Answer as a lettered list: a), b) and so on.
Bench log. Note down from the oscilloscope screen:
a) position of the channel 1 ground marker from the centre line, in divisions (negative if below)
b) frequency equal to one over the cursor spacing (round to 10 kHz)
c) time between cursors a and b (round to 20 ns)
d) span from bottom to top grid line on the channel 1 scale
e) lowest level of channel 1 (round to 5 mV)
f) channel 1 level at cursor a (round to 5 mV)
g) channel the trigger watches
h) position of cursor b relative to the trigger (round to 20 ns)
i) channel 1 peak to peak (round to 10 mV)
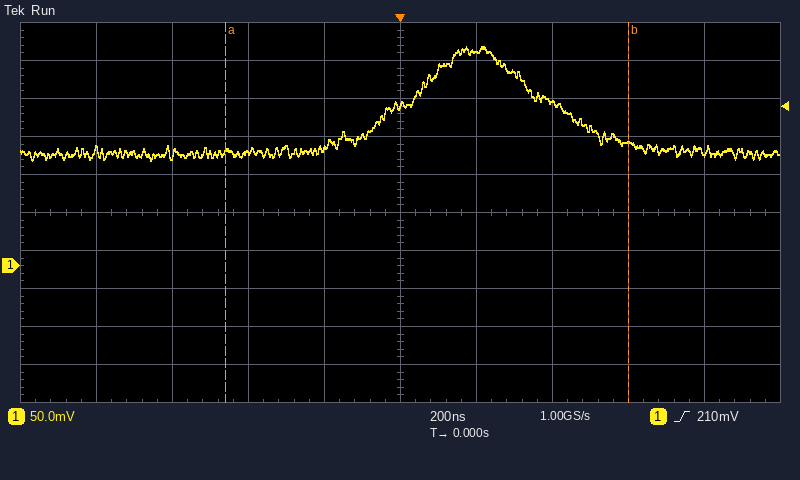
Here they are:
a) -1.4 div
b) 940 kHz
c) 1.06 µs
d) 500 mV
e) 140 mV
f) 150 mV
g) channel 1
h) +600 ns
i) 150 mV
